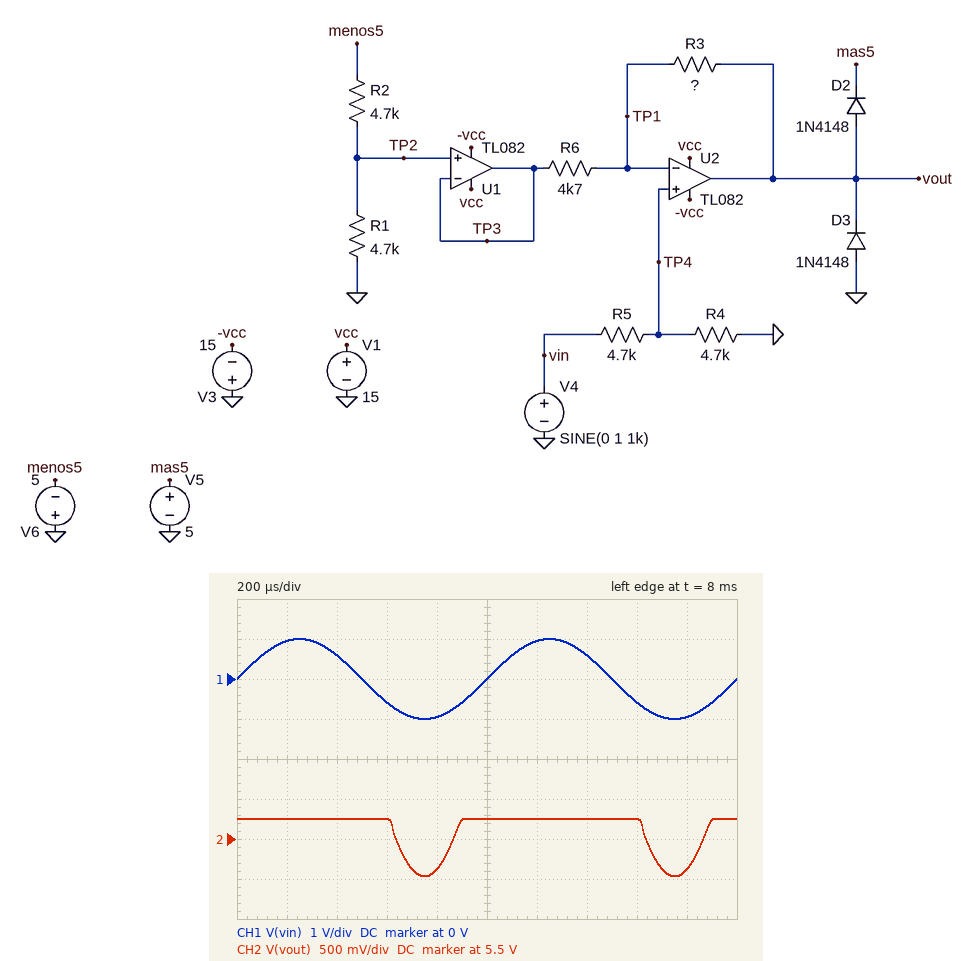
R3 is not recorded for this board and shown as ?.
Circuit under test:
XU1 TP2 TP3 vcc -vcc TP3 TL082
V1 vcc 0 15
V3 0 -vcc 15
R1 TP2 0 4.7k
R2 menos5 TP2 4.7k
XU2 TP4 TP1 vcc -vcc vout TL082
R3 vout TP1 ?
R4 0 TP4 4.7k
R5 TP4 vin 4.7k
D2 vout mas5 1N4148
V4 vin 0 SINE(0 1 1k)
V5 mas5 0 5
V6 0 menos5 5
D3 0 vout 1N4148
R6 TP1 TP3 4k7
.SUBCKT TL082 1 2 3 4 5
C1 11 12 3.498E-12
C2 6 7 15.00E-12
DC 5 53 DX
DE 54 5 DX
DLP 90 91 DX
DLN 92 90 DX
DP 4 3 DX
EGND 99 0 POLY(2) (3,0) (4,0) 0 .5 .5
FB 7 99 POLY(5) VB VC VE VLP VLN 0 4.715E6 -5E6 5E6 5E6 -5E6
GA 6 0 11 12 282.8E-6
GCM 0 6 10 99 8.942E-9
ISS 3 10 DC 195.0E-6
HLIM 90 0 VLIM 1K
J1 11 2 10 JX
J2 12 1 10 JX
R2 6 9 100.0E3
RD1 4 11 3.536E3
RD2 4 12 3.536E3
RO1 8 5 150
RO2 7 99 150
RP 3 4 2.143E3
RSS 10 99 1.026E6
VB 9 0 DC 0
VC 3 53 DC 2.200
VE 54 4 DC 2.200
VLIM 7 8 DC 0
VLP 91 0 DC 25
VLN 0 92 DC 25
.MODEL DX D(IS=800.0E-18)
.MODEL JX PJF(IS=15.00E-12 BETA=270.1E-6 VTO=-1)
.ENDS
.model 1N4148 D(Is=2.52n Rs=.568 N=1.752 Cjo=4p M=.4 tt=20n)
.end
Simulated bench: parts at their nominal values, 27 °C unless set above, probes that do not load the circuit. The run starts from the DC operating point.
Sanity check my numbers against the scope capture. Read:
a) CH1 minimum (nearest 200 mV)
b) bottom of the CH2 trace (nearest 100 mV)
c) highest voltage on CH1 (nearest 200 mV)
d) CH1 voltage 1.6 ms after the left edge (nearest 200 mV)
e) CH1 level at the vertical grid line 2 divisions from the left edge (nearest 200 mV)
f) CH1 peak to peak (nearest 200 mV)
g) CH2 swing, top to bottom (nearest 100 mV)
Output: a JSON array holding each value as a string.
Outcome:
["-1.0 V", "5.0 V", "1.0 V", "-600 mV", "600 mV", "2.0 V", "700 mV"]
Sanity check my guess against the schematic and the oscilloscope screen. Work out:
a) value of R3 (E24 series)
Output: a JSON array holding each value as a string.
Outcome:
["13 kΩ"]
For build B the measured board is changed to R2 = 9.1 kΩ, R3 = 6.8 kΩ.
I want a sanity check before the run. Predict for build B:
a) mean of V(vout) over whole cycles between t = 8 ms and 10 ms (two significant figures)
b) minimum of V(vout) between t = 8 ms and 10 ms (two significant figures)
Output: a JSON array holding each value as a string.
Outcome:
["2.5 V", "1.2 V"]
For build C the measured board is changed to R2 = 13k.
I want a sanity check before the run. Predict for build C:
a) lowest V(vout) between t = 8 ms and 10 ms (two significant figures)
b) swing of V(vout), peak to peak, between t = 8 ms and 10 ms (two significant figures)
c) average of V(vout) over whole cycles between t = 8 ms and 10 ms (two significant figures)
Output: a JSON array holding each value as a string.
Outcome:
["1.8 V", "3.8 V", "3.7 V"]
